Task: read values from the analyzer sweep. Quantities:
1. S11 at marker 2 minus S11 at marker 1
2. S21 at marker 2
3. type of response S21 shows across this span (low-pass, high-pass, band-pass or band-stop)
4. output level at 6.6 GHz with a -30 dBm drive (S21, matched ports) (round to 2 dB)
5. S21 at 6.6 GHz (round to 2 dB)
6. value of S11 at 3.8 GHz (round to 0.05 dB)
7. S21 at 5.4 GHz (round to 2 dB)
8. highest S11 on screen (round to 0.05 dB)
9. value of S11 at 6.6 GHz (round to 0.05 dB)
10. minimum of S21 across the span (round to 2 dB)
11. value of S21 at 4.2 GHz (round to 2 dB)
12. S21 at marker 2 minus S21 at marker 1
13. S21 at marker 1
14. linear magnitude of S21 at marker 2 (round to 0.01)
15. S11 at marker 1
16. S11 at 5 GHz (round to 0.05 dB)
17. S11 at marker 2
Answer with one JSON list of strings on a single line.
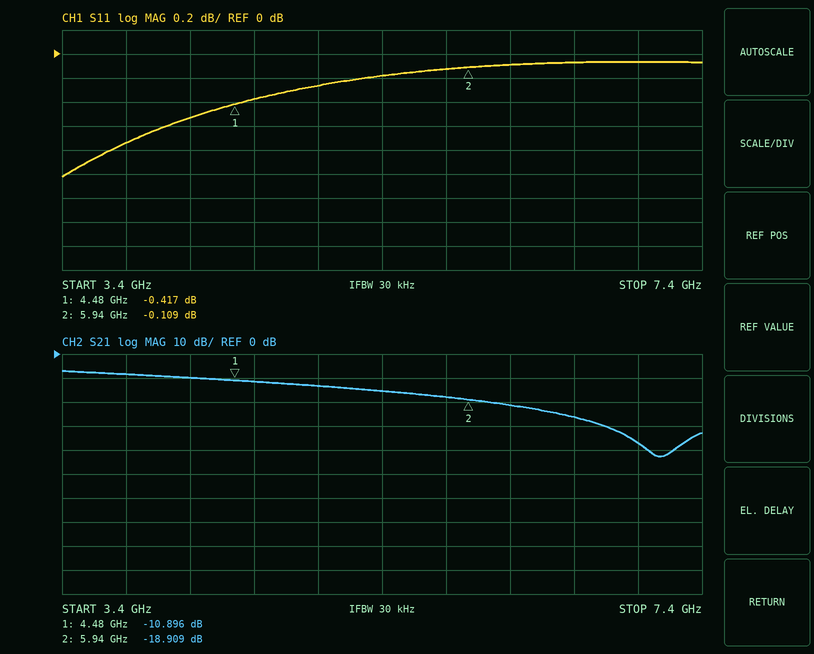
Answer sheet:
["0.308 dB", "-18.909 dB", "low-pass", "-56 dBm", "-26 dB", "-0.75 dB", "-16 dB", "-0.05 dB", "-0.05 dB", "-42 dB", "-10 dB", "-8.013 dB", "-10.896 dB", "0.11", "-0.417 dB", "-0.25 dB", "-0.109 dB"]
